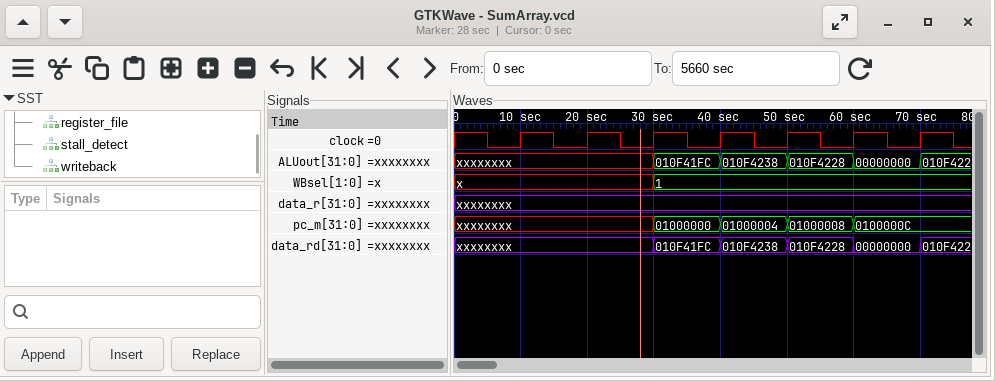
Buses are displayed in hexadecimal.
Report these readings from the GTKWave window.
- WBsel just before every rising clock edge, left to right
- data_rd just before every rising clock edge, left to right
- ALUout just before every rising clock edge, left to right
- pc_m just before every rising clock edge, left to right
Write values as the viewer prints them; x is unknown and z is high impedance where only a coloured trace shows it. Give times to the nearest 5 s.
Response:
x, x, x, 1, 1, 1, 1
xxxxxxxx, xxxxxxxx, xxxxxxxx, 010F41FC, 010F4238, 010F4228, 00000000
xxxxxxxx, xxxxxxxx, xxxxxxxx, 010F41FC, 010F4238, 010F4228, 00000000
xxxxxxxx, xxxxxxxx, xxxxxxxx, 01000000, 01000004, 01000008, 0100000C
